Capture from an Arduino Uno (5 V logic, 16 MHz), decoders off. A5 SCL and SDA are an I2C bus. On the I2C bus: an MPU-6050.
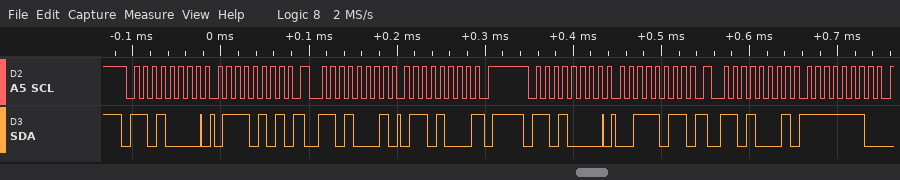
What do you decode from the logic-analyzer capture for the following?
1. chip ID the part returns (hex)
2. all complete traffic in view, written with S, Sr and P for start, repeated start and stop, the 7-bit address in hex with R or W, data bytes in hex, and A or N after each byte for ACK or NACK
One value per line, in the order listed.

0x68
S 68W A 75 A Sr 68R A 68 N P S 68W A 3B A Sr 68R A FE A
